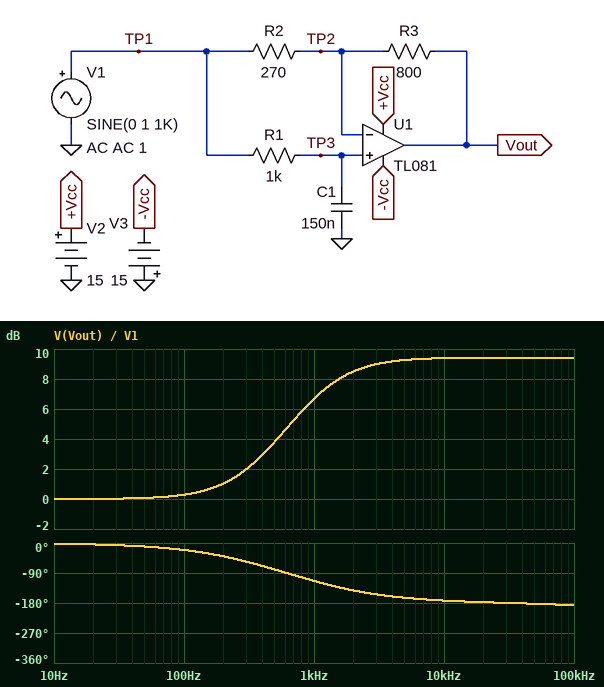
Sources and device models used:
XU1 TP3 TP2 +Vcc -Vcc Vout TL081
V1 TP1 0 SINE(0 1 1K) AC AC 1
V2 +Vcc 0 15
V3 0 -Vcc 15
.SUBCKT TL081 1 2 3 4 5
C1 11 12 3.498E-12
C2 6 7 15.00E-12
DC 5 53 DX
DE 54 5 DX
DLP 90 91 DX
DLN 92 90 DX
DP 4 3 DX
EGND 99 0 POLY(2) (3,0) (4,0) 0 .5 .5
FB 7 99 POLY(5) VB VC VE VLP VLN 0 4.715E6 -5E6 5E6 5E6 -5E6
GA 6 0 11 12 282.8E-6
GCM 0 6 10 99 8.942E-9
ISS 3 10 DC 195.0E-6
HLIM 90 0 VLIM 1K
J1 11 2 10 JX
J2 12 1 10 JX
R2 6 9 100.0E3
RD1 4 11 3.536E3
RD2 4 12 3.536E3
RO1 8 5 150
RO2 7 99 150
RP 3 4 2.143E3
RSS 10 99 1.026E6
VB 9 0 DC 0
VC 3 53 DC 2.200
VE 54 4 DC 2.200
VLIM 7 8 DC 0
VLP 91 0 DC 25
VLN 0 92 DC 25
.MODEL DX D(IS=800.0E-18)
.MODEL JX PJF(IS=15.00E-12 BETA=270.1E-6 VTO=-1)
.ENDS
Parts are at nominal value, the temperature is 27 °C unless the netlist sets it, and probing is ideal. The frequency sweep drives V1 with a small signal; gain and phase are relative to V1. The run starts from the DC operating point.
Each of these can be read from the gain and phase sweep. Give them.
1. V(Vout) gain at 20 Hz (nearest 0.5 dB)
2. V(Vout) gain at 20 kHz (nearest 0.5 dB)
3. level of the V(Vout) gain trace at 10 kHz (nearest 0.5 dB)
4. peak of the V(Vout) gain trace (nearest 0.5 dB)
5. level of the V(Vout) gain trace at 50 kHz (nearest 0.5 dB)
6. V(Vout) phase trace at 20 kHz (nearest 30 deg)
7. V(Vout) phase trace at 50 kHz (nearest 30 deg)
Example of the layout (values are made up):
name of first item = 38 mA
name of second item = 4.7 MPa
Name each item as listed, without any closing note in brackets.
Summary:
V(Vout) gain at 20 Hz = 0 dB
V(Vout) gain at 20 kHz = 9.5 dB
level of the V(Vout) gain trace at 10 kHz = 9.5 dB
peak of the V(Vout) gain trace = 9.5 dB
level of the V(Vout) gain trace at 50 kHz = 9.5 dB
V(Vout) phase trace at 20 kHz = -180 deg
V(Vout) phase trace at 50 kHz = -180 deg
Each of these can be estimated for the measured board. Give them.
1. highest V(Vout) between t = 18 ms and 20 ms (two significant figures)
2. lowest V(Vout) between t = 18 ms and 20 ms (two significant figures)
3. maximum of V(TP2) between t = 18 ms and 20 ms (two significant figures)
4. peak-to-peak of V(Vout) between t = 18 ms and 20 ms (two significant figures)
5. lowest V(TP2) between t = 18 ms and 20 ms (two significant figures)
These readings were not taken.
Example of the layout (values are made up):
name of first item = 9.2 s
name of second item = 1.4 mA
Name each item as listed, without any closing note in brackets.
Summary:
highest V(Vout) between t = 18 ms and 20 ms = 2.2 V
lowest V(Vout) between t = 18 ms and 20 ms = -2.2 V
maximum of V(TP2) between t = 18 ms and 20 ms = 730 mV
peak-to-peak of V(Vout) between t = 18 ms and 20 ms = 4.3 V
lowest V(TP2) between t = 18 ms and 20 ms = -730 mV
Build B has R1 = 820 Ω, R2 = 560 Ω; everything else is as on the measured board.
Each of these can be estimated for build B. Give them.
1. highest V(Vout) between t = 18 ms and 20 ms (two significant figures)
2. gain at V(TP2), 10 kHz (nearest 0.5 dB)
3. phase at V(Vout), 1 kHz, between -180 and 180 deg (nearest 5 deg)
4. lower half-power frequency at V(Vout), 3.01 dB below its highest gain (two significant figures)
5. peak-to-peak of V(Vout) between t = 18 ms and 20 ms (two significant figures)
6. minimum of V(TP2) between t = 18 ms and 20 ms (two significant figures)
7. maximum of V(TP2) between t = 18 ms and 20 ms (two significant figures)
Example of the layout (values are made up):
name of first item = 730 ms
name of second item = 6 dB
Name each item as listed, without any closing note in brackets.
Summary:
highest V(Vout) between t = 18 ms and 20 ms = 1.2 V
gain at V(TP2), 10 kHz = -18.0 dB
phase at V(Vout), 1 kHz, between -180 and 180 deg = -85 deg
lower half-power frequency at V(Vout), 3.01 dB below its highest gain = 180 Hz
peak-to-peak of V(Vout) between t = 18 ms and 20 ms = 2.4 V
minimum of V(TP2) between t = 18 ms and 20 ms = -790 mV
maximum of V(TP2) between t = 18 ms and 20 ms = 790 mV
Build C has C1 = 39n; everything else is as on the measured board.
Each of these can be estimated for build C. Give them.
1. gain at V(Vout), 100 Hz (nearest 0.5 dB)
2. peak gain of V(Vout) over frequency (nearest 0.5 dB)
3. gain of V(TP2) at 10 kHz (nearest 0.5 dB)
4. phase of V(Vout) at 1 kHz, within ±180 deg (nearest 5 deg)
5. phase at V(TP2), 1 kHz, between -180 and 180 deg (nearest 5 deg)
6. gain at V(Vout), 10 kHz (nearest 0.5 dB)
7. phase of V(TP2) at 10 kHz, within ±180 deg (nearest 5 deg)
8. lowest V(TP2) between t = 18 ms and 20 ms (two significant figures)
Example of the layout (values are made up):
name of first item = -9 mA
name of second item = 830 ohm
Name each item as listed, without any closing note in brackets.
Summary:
gain at V(Vout), 100 Hz = 0 dB
peak gain of V(Vout) over frequency = 9.5 dB
gain of V(TP2) at 10 kHz = -8.5 dB
phase of V(Vout) at 1 kHz, within ±180 deg = -50 deg
phase at V(TP2), 1 kHz, between -180 and 180 deg = -15 deg
gain at V(Vout), 10 kHz = 9.0 dB
phase of V(TP2) at 10 kHz, within ±180 deg = -70 deg
lowest V(TP2) between t = 18 ms and 20 ms = -970 mV
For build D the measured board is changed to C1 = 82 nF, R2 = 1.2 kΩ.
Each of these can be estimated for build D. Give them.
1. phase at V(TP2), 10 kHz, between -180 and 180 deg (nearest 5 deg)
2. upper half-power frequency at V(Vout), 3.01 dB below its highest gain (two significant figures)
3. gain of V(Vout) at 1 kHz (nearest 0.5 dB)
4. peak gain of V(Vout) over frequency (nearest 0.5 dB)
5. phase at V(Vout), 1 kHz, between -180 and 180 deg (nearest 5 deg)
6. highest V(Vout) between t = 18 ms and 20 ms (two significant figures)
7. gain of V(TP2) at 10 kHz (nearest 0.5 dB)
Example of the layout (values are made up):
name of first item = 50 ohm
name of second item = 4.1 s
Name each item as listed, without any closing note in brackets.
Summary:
phase at V(TP2), 10 kHz, between -180 and 180 deg = -80 deg
upper half-power frequency at V(Vout), 3.01 dB below its highest gain = 5.8 kHz
gain of V(Vout) at 1 kHz = -0.5 dB
peak gain of V(Vout) over frequency = 0 dB
phase at V(Vout), 1 kHz, between -180 and 180 deg = -45 deg
highest V(Vout) between t = 18 ms and 20 ms = 940 mV
gain of V(TP2) at 10 kHz = -14.5 dB
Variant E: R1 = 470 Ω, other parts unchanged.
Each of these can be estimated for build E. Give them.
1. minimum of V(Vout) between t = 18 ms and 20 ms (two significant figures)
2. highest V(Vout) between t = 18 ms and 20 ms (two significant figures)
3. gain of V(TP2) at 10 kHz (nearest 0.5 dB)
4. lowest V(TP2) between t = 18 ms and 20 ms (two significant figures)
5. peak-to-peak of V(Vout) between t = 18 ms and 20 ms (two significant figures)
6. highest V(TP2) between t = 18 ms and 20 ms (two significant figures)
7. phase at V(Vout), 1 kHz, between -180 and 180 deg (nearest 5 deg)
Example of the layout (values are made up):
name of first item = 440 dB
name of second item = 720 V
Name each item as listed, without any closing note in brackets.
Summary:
minimum of V(Vout) between t = 18 ms and 20 ms = -1.5 V
highest V(Vout) between t = 18 ms and 20 ms = 1.5 V
gain of V(TP2) at 10 kHz = -13.5 dB
lowest V(TP2) between t = 18 ms and 20 ms = -910 mV
peak-to-peak of V(Vout) between t = 18 ms and 20 ms = 3.0 V
highest V(TP2) between t = 18 ms and 20 ms = 910 mV
phase at V(Vout), 1 kHz, between -180 and 180 deg = -75 deg
